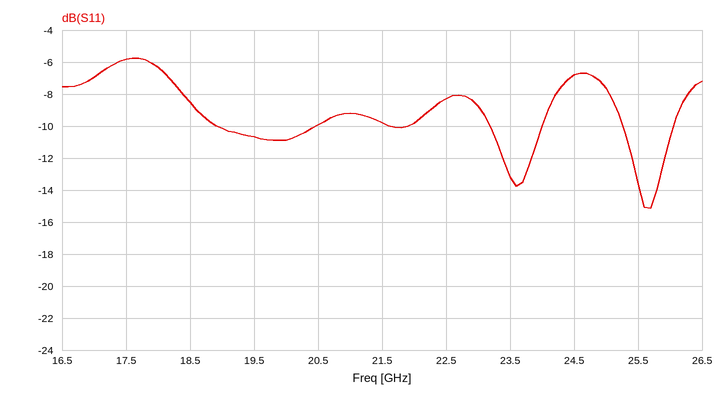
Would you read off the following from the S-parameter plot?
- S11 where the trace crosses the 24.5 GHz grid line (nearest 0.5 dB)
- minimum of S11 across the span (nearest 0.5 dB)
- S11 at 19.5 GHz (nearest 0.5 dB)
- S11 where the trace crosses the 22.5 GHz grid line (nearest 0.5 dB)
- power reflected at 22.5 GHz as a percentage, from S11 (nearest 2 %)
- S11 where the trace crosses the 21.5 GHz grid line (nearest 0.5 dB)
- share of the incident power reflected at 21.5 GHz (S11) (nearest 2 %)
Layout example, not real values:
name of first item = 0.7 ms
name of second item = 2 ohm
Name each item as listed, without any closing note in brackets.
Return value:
S11 where the trace crosses the 24.5 GHz grid line = -7.0 dB
minimum of S11 across the span = -15.0 dB
S11 at 19.5 GHz = -10.5 dB
S11 where the trace crosses the 22.5 GHz grid line = -8.5 dB
power reflected at 22.5 GHz as a percentage, from S11 = 14 %
S11 where the trace crosses the 21.5 GHz grid line = -10.0 dB
share of the incident power reflected at 21.5 GHz (S11) = 10 %
